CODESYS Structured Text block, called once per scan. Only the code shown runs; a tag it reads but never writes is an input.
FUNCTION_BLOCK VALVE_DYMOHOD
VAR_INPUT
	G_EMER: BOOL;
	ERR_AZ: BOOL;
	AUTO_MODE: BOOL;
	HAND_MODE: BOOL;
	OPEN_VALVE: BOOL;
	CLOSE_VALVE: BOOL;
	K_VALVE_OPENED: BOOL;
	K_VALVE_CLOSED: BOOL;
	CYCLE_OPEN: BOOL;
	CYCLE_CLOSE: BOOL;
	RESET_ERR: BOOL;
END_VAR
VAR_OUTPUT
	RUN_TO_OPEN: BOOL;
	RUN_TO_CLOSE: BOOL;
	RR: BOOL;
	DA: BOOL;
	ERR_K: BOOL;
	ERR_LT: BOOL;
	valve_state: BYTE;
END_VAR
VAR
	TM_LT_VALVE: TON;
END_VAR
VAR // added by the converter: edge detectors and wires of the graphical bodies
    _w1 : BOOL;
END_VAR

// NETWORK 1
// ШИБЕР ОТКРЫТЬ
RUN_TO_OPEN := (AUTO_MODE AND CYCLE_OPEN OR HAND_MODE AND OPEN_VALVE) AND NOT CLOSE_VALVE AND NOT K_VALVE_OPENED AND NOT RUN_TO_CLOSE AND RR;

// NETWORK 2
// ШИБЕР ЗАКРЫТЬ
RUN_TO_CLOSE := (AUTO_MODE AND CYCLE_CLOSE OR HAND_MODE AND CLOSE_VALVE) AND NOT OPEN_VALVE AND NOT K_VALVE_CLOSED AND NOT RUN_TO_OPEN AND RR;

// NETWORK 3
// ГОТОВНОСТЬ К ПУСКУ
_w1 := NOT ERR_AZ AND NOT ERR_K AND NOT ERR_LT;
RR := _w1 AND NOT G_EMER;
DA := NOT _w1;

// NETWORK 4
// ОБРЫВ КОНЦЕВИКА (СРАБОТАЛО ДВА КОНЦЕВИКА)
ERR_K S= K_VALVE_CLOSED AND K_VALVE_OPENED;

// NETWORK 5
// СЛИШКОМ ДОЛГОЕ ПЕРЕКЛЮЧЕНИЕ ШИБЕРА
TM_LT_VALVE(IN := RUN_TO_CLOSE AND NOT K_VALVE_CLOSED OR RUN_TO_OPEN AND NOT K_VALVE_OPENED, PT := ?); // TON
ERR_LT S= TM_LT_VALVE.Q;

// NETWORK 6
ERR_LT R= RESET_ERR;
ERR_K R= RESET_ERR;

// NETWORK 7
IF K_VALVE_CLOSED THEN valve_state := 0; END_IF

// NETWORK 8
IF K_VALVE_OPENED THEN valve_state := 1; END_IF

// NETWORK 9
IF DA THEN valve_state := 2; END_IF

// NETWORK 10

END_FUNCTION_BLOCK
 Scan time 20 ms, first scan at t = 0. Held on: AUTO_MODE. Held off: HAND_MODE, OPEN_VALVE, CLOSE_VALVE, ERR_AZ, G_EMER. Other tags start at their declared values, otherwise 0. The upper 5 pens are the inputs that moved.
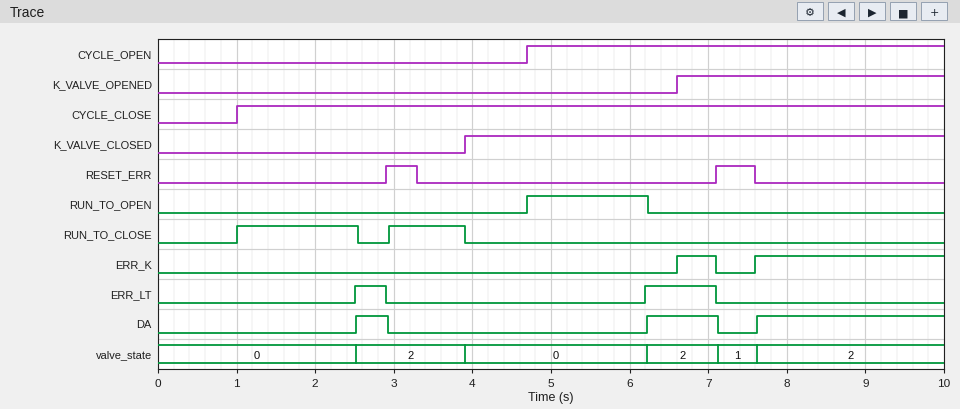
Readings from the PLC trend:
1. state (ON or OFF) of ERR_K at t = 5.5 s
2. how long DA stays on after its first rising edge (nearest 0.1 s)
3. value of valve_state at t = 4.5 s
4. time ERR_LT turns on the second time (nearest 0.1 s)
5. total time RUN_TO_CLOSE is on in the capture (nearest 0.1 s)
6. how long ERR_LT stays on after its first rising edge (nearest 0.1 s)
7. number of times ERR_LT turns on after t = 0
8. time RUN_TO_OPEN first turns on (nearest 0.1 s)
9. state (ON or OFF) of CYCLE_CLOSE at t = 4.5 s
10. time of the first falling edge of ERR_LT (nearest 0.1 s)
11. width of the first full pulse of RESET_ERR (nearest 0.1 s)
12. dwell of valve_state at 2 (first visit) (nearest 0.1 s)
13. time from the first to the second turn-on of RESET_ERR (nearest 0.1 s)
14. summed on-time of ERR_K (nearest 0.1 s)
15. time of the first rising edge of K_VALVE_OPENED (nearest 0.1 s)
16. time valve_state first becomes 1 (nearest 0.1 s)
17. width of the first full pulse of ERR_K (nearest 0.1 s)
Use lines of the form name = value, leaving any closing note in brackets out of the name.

state (ON or OFF) of ERR_K at t = 5.5 s = OFF
how long DA stays on after its first rising edge = 0.4 s
value of valve_state at t = 4.5 s = 0
time ERR_LT turns on the second time = 6.2 s
total time RUN_TO_CLOSE is on in the capture = 2.5 s
how long ERR_LT stays on after its first rising edge = 0.4 s
number of times ERR_LT turns on after t = 0 = 2
time RUN_TO_OPEN first turns on = 4.7 s
state (ON or OFF) of CYCLE_CLOSE at t = 4.5 s = ON
time of the first falling edge of ERR_LT = 2.9 s
width of the first full pulse of RESET_ERR = 0.4 s
dwell of valve_state at 2 (first visit) = 1.4 s
time from the first to the second turn-on of RESET_ERR = 4.2 s
summed on-time of ERR_K = 2.9 s
time of the first rising edge of K_VALVE_OPENED = 6.6 s
time valve_state first becomes 1 = 7.1 s
width of the first full pulse of ERR_K = 0.5 s
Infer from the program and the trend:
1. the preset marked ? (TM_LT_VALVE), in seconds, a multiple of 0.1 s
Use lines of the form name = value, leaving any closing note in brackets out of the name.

the preset marked ? (TM_LT_VALVE), in seconds, a multiple of 0.1 s = 1.5 s
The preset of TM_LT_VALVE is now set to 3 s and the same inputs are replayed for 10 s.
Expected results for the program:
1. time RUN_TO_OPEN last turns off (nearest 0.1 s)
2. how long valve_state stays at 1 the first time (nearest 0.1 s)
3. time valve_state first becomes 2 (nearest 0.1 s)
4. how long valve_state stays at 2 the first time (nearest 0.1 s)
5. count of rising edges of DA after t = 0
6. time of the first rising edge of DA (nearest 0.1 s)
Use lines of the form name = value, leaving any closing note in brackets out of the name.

time RUN_TO_OPEN last turns off = 6.6 s
how long valve_state stays at 1 the first time = 0.0 s
time valve_state first becomes 2 = 6.6 s
how long valve_state stays at 2 the first time = 0.5 s
count of rising edges of DA after t = 0 = 2
time of the first rising edge of DA = 6.6 s
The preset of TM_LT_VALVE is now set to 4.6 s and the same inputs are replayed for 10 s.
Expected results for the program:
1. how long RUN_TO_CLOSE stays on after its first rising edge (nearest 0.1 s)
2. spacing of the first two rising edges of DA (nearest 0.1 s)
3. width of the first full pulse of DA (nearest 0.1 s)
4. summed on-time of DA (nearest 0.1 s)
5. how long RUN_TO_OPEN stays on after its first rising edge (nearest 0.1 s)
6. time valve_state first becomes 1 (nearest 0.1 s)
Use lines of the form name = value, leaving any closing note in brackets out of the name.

how long RUN_TO_CLOSE stays on after its first rising edge = 2.9 s
spacing of the first two rising edges of DA = 1.0 s
width of the first full pulse of DA = 0.5 s
summed on-time of DA = 2.9 s
how long RUN_TO_OPEN stays on after its first rising edge = 1.9 s
time valve_state first becomes 1 = 6.6 s
